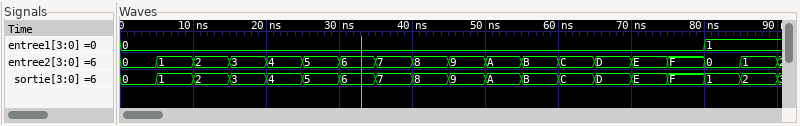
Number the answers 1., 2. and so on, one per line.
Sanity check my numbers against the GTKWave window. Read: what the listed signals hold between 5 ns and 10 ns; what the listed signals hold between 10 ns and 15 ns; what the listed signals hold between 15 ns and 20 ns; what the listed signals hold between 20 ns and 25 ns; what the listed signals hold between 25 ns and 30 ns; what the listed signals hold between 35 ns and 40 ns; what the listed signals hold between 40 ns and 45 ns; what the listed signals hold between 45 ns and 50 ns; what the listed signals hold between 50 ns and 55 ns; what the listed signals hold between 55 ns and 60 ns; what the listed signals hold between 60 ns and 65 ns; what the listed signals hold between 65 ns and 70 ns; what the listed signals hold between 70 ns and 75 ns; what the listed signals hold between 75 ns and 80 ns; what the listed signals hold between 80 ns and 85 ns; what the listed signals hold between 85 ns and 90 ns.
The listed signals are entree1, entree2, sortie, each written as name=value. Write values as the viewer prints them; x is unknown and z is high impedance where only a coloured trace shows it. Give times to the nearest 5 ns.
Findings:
1. entree1=0, entree2=1, sortie=1
2. entree1=0, entree2=2, sortie=2
3. entree1=0, entree2=3, sortie=3
4. entree1=0, entree2=4, sortie=4
5. entree1=0, entree2=5, sortie=5
6. entree1=0, entree2=7, sortie=7
7. entree1=0, entree2=8, sortie=8
8. entree1=0, entree2=9, sortie=9
9. entree1=0, entree2=A, sortie=A
10. entree1=0, entree2=B, sortie=B
11. entree1=0, entree2=C, sortie=C
12. entree1=0, entree2=D, sortie=D
13. entree1=0, entree2=E, sortie=E
14. entree1=0, entree2=F, sortie=F
15. entree1=1, entree2=0, sortie=1
16. entree1=1, entree2=1, sortie=2
